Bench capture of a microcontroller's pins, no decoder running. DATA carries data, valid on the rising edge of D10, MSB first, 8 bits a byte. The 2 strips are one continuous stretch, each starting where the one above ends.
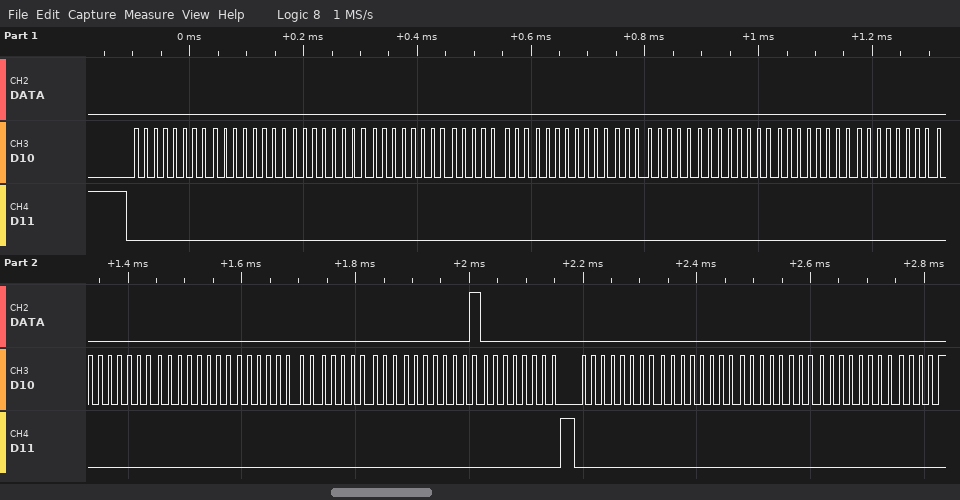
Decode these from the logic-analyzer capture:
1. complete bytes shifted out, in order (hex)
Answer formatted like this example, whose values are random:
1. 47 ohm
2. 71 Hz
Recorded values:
1. 0x00 0x00 0x00 0x00 0x00 0x00 0x00 0x00 0x00 0x00 0x00 0x00 0x00 0x00 0x01 0x00 0x00 0x00 0x00 0x00
